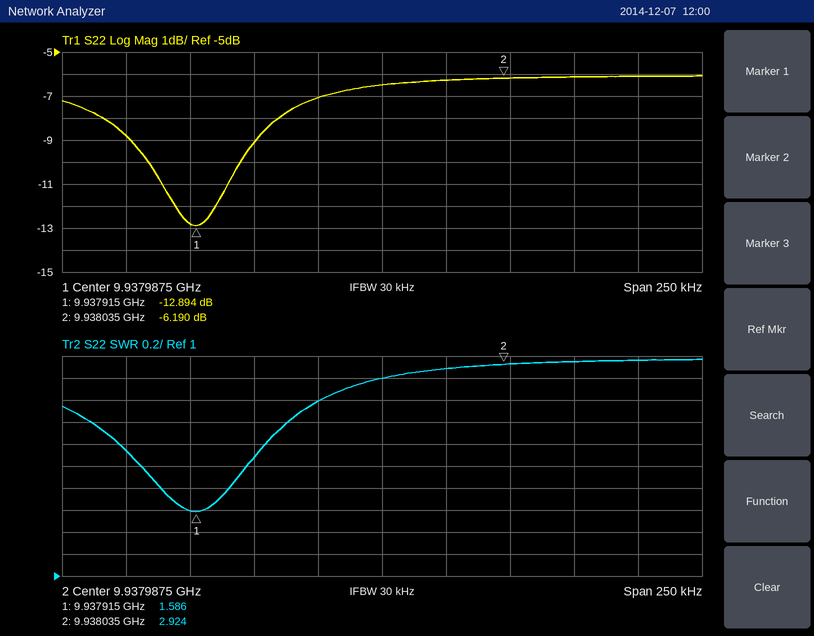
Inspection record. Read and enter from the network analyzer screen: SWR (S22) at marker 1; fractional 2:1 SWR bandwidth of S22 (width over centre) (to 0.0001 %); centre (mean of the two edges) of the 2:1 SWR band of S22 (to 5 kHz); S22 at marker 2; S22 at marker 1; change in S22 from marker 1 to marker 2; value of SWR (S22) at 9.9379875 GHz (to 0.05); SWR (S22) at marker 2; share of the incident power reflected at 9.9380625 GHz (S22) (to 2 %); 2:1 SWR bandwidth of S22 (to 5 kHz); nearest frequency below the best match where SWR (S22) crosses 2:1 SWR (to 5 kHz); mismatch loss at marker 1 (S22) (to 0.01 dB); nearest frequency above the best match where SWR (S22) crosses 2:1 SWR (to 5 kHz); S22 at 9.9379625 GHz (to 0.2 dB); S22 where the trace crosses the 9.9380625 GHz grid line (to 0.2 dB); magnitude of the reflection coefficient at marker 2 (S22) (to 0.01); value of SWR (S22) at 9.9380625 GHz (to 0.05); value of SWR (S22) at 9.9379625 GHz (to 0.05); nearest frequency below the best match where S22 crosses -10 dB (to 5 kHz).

1.586
0.0004 %
9.937915 GHz
-6.190 dB
-12.894 dB
6.704 dB
2.80
2.924
24 %
40 kHz
9.937895 GHz
0.23 dB
9.937935 GHz
-7.0 dB
-6.2 dB
0.49
2.95
2.60
9.937895 GHz
